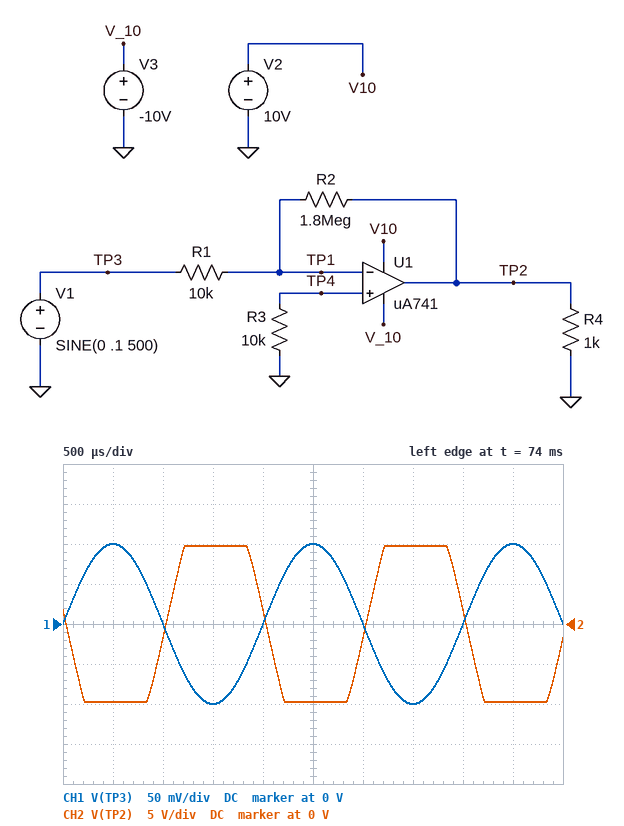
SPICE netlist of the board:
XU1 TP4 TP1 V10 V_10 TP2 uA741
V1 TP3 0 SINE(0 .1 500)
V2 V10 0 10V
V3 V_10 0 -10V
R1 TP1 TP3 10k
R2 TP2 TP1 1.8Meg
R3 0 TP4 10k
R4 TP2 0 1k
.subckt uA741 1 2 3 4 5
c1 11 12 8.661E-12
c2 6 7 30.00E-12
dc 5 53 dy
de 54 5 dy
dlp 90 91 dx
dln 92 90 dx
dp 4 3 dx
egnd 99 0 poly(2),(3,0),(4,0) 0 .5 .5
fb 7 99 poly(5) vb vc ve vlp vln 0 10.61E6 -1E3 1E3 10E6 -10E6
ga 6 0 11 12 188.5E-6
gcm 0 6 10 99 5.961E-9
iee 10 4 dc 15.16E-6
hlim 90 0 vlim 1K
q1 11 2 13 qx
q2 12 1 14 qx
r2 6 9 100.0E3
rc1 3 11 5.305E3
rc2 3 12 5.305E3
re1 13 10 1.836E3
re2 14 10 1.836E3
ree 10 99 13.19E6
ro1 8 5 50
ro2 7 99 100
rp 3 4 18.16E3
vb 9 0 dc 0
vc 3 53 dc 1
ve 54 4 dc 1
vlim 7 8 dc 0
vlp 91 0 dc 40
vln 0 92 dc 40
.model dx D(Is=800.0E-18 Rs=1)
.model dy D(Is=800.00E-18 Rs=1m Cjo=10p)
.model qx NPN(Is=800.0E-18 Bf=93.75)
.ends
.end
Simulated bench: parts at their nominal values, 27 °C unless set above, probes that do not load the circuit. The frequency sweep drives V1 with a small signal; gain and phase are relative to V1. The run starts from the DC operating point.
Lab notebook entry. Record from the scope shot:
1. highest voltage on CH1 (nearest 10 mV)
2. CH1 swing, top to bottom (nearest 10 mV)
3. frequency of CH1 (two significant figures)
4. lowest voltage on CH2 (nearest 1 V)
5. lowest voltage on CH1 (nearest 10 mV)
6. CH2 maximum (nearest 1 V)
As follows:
100 mV
200 mV
500 Hz
-10 V
-100 mV
10 V
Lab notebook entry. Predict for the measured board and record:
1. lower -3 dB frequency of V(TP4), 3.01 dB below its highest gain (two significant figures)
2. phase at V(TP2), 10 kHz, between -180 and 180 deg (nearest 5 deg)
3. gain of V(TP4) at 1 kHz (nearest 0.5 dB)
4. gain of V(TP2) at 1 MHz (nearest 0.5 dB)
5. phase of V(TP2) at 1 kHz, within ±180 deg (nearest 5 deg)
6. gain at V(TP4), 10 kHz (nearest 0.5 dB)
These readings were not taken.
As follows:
5.2 kHz
115 deg
-54.5 dB
-2.0 dB
170 deg
-41.0 dB
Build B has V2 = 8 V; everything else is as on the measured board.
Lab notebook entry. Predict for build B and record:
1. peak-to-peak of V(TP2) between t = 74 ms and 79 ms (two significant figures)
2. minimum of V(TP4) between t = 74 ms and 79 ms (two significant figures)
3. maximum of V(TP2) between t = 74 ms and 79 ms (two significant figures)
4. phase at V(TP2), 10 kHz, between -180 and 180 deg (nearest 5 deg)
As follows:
18 V
-1.3 mV
7.8 V
115 deg
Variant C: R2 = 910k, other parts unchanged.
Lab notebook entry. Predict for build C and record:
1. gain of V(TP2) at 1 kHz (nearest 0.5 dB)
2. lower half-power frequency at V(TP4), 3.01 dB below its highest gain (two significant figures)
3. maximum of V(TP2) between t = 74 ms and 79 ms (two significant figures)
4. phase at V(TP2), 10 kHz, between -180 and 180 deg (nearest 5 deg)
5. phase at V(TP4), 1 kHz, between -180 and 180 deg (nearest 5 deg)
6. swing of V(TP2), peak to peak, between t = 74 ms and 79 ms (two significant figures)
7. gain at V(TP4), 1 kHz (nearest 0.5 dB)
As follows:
39.0 dB
10 kHz
9.1 V
135 deg
85 deg
18 V
-60.5 dB
